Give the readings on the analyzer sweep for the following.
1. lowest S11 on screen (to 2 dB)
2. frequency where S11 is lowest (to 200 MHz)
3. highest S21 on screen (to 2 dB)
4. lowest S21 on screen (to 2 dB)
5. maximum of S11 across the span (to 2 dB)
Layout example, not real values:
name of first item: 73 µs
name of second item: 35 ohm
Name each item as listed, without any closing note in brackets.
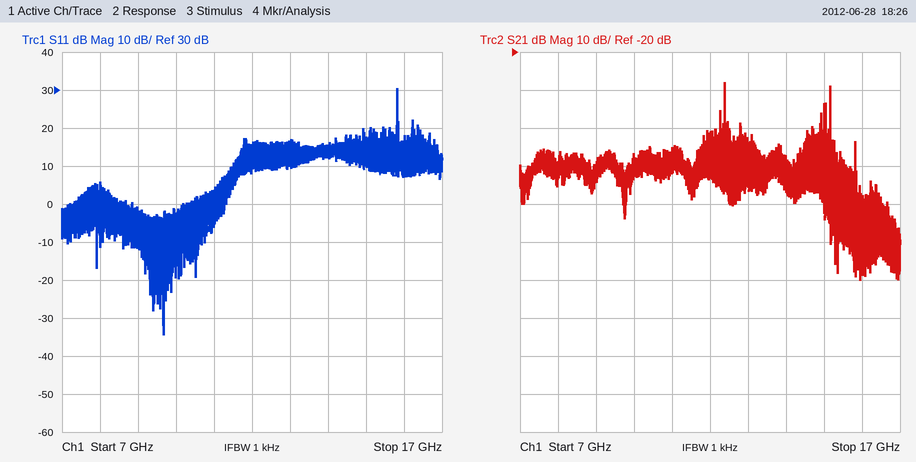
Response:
lowest S11 on screen: -34 dB
frequency where S11 is lowest: 9.6 GHz
highest S21 on screen: -28 dB
lowest S21 on screen: -80 dB
maximum of S11 across the span: 30 dB
